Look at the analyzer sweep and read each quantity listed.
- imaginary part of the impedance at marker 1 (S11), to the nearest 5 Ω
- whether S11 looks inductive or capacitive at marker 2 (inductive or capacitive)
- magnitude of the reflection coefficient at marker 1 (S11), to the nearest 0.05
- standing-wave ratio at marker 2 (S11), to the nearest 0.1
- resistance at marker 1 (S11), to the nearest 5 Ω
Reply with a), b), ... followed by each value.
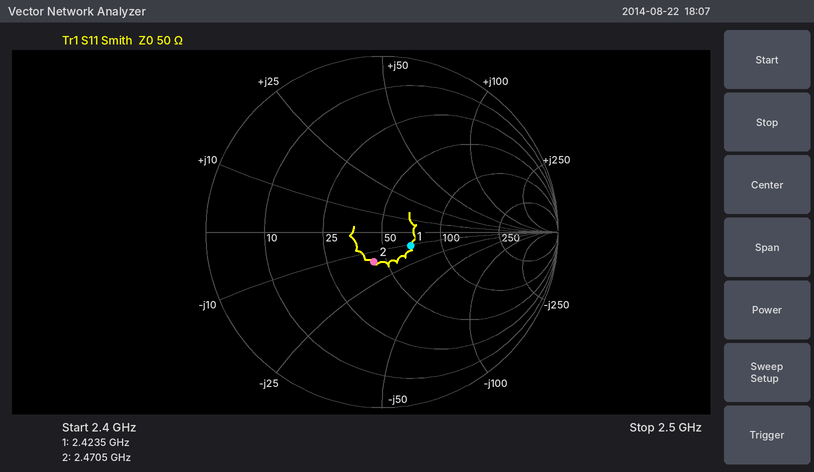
a) -10 Ω
b) capacitive
c) 0.20
d) 1.4
e) 70 Ω
